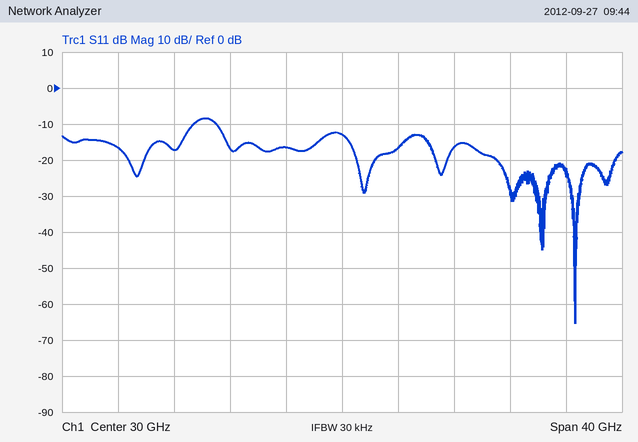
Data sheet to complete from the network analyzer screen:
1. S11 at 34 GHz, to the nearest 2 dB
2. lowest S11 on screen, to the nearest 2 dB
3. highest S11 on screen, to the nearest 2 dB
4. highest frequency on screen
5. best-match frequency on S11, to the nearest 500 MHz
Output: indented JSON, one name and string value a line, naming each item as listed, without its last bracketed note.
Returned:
{
  "S11 at 34 GHz, to the nearest 2 dB": "-16 dB",
  "lowest S11 on screen, to the nearest 2 dB": "-66 dB",
  "highest S11 on screen, to the nearest 2 dB": "-8 dB",
  "highest frequency on screen": "50 GHz",
  "best-match frequency on S11, to the nearest 500 MHz": "46.5 GHz"
}
